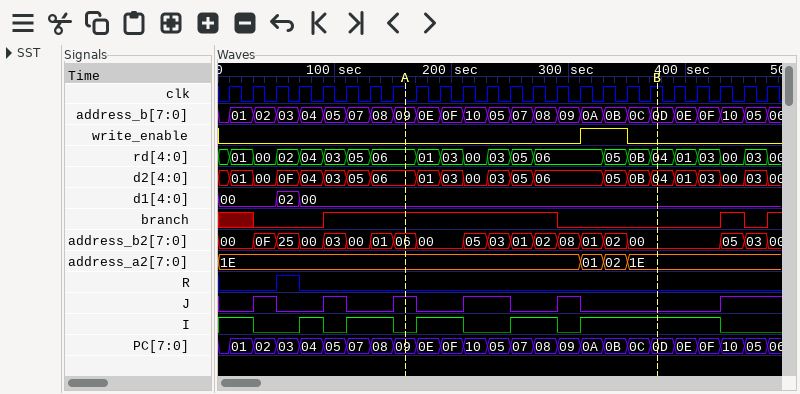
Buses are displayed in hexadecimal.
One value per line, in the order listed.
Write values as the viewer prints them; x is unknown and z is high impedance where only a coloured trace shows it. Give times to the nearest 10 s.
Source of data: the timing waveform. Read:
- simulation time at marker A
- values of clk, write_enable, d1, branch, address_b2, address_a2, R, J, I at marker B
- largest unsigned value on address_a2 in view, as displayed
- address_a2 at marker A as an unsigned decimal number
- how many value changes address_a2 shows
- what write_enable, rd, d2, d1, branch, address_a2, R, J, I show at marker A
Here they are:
160 s
clk=1, write_enable=0, d1=00, branch=0, address_b2=00, address_a2=1E, R=0, J=0, I=1
1E
30
3
write_enable=0, rd=06, d2=06, d1=00, branch=1, address_a2=1E, R=0, J=1, I=0
